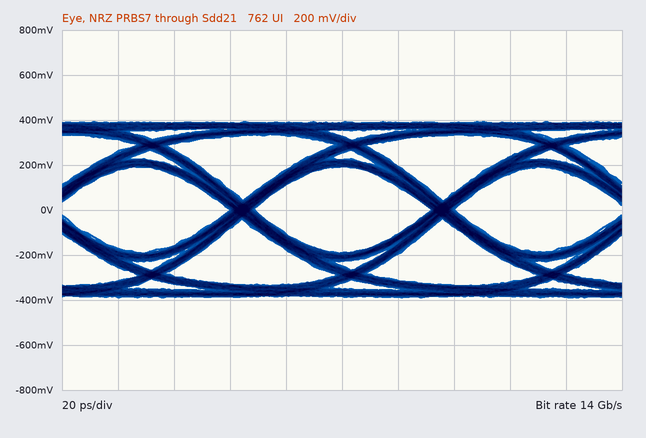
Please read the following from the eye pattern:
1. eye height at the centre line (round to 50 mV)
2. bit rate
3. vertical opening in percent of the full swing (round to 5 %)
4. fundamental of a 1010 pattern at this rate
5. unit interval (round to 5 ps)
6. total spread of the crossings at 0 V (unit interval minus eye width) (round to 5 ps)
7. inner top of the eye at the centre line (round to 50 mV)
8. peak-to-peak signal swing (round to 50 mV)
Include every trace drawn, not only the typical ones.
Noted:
400 mV
14 Gb/s
50 %
7 GHz
70 ps
10 ps
200 mV
800 mV
